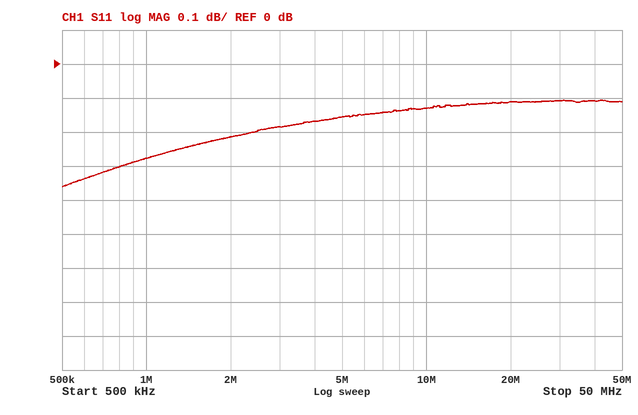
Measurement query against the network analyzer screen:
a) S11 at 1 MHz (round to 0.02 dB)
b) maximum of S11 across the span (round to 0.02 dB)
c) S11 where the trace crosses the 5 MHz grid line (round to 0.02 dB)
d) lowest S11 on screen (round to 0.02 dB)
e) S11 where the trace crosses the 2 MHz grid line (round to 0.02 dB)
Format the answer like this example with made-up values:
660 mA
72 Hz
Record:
-0.28 dB
-0.10 dB
-0.16 dB
-0.36 dB
-0.22 dB
